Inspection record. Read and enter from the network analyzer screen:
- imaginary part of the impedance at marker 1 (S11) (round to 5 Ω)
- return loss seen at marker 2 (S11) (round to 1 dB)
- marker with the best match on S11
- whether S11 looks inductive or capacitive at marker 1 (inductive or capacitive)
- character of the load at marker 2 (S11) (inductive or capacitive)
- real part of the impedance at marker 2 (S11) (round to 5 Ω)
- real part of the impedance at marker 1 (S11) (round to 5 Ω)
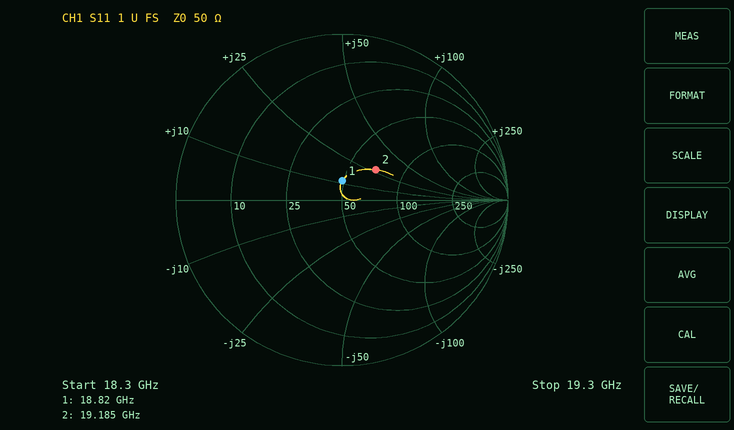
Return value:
+10 Ω
11 dB
marker 1
inductive
inductive
70 Ω
50 Ω
